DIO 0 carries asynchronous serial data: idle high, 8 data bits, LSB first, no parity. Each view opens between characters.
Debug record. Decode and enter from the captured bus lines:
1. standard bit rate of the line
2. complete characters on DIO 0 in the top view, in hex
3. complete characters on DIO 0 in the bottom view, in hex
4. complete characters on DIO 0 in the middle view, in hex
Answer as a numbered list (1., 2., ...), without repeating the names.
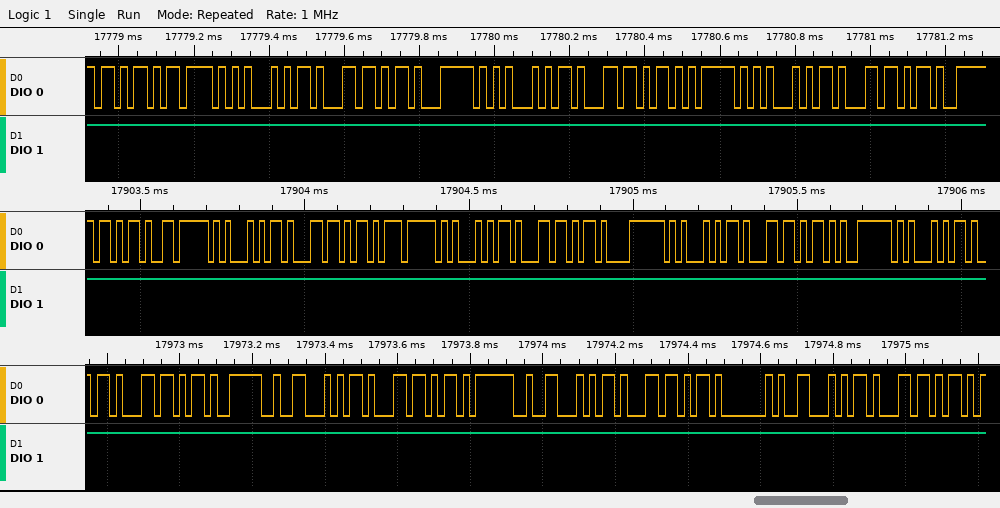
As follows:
1. 57600 baud
2. 6B, 7B, 45, 8B, 6B, 7C, 45, 8B, 6B, 7D, 45, 8B, 6B
3. 8B, 6B, 3E, 46, 8B, 6B, 3F, 46, 8B, 6B, 40, 46, 8B, 6B
4. 6B, F6, 45, 8B, 6B, F7, 45, 8B, 6B, F8, 45, 8B, 6B, F9, 45
